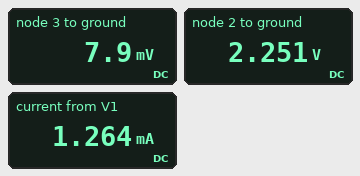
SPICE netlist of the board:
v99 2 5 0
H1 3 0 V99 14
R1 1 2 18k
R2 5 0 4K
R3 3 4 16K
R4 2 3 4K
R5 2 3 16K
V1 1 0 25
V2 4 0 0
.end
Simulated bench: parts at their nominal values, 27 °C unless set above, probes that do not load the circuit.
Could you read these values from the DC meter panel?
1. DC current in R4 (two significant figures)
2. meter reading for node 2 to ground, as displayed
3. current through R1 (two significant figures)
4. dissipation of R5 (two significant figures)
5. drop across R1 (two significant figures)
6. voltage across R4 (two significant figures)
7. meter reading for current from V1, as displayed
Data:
560 µA
2.251 V
1.3 mA
310 µW
23 V
2.2 V
1.264 mA
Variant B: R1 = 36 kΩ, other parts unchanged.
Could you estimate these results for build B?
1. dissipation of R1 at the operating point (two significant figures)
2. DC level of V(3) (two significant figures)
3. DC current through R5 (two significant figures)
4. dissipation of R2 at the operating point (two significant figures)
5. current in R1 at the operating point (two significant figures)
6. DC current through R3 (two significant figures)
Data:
16 mW
4.1 mV
73 µA
350 µW
660 µA
260 nA
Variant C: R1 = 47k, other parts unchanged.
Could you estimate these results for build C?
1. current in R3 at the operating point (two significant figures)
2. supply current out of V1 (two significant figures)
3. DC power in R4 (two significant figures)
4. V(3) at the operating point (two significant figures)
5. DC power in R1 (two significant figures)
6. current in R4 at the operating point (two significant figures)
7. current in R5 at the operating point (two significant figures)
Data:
200 nA
510 µA
210 µW
3.2 mV
12 mW
230 µA
57 µA
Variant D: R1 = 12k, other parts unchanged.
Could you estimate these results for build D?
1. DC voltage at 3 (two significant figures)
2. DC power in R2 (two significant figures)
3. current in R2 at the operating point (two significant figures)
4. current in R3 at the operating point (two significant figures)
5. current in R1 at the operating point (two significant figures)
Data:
11 mV
2.6 mW
810 µA
710 nA
1.8 mA
